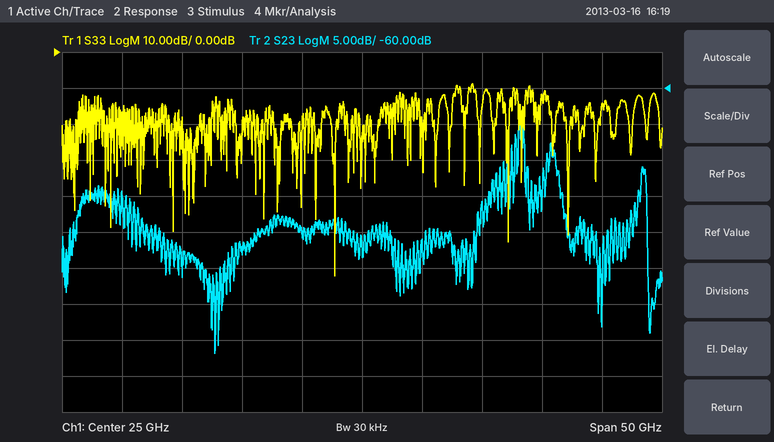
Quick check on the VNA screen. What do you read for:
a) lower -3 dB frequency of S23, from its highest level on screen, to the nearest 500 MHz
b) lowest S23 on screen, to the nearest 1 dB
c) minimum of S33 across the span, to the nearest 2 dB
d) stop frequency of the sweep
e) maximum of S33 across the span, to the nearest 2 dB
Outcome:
38.0 GHz
-97 dB
-62 dB
50 GHz
-8 dB
